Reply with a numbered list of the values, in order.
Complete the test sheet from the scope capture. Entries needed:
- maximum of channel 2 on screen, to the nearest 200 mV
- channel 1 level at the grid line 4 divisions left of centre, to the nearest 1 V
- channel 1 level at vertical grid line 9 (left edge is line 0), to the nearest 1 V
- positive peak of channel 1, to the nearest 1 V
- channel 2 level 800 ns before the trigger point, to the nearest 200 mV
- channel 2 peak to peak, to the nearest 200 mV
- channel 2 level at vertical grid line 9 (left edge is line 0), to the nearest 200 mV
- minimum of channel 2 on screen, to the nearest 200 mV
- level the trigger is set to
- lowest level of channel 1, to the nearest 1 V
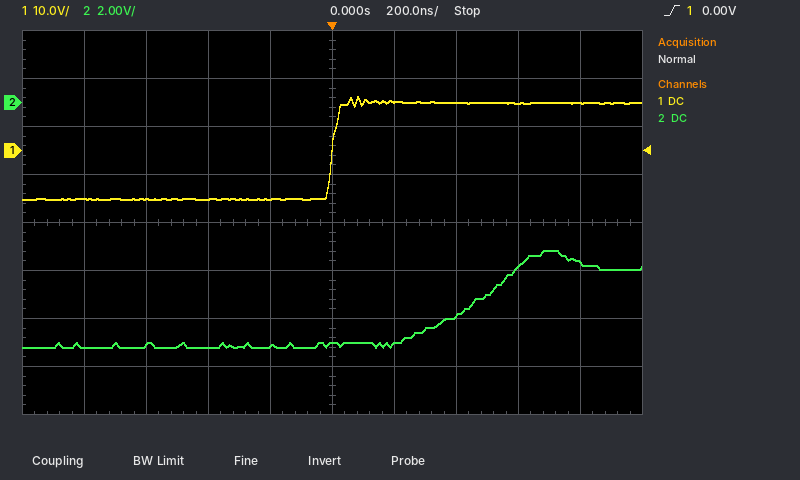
1. -6.2 V
2. -10 V
3. 10 V
4. 11 V
5. -10.2 V
6. 4.0 V
7. -6.6 V
8. -10.2 V
9. 0.00 V
10. -10 V
